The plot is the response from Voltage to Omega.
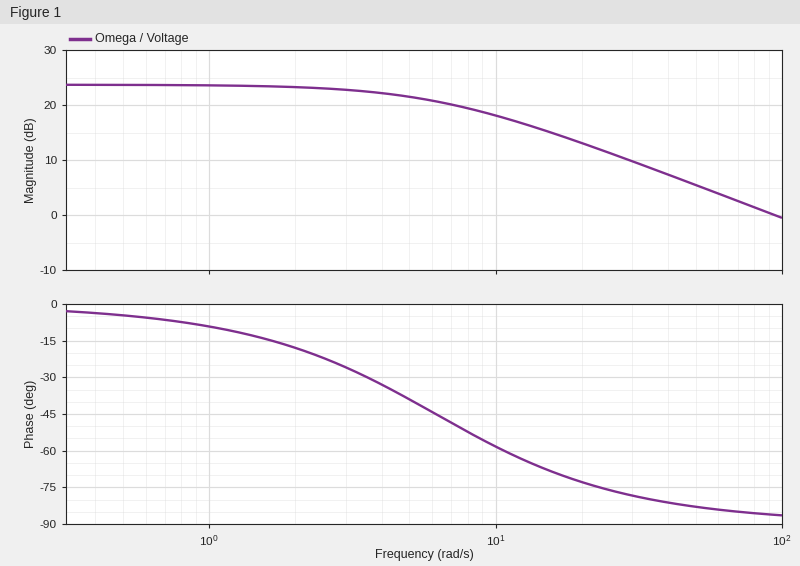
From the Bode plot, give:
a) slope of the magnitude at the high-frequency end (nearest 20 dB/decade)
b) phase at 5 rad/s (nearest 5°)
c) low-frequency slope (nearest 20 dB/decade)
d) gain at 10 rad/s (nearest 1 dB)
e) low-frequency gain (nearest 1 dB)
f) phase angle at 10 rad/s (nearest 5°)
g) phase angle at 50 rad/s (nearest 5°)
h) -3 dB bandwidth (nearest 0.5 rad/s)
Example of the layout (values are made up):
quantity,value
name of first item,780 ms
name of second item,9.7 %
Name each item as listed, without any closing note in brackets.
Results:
quantity,value
slope of the magnitude at the high-frequency end,-20 dB/decade
phase at 5 rad/s,-40°
low-frequency slope,0 dB/decade
gain at 10 rad/s,18 dB
low-frequency gain,24 dB
phase angle at 10 rad/s,-60°
phase angle at 50 rad/s,-85°
-3 dB bandwidth,6.0 rad/s
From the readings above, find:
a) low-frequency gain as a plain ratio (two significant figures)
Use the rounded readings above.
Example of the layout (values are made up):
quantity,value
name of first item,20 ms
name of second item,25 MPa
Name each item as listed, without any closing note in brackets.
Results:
quantity,value
low-frequency gain as a plain ratio,16
